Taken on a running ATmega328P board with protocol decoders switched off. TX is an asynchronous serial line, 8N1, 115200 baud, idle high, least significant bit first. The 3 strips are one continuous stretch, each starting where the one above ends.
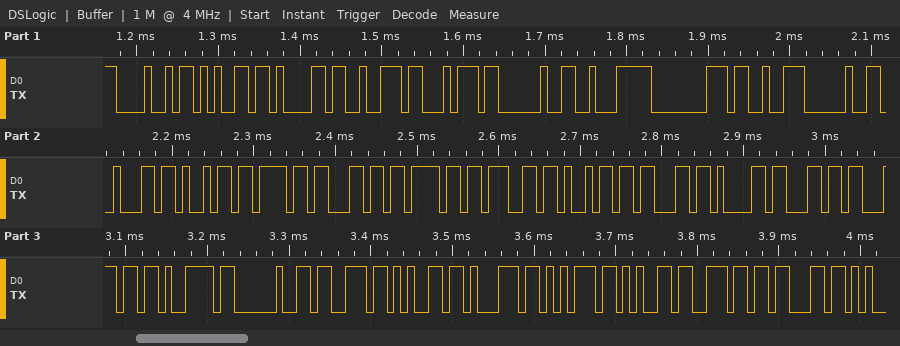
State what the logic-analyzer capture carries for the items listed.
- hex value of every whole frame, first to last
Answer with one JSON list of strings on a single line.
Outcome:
["48 65 61 72 74 20 E2 80 93 20 62 69 6F 6C 6F 67 69 63 61 6C 6C 79 20 73 65 71 75 65 6E 63"]
